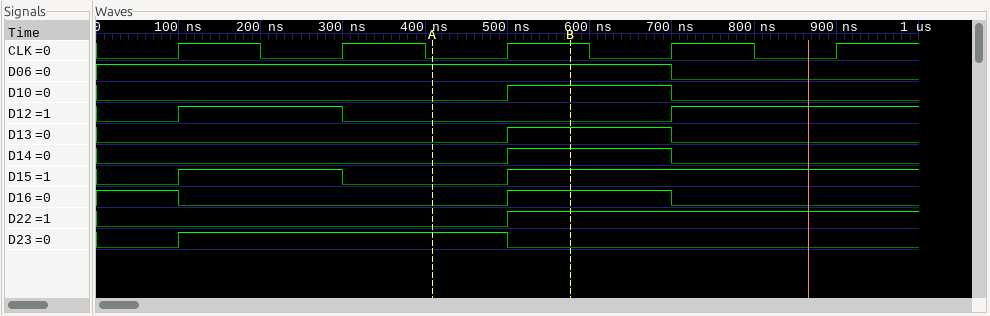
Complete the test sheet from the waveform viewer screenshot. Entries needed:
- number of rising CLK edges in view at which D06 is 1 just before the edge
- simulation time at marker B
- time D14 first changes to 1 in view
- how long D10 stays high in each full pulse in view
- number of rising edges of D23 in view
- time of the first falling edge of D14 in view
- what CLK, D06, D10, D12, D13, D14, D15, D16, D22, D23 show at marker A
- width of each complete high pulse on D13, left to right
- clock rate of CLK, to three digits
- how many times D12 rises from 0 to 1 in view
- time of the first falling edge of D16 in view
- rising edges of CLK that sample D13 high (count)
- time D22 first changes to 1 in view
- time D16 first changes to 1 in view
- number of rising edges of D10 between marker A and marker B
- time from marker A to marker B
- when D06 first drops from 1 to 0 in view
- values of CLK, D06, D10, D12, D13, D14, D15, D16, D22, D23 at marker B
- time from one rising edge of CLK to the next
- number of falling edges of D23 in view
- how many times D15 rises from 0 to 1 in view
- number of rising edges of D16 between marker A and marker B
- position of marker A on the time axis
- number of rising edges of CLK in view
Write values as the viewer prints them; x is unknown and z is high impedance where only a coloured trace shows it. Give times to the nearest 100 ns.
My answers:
4
600 ns
500 ns
200 ns
1
700 ns
CLK=0, D06=1, D10=0, D12=0, D13=0, D14=0, D15=0, D16=0, D22=0, D23=1
200 ns
5.00 MHz
2
100 ns
1
500 ns
500 ns
1
200 ns
700 ns
CLK=1, D06=1, D10=1, D12=0, D13=1, D14=1, D15=1, D16=1, D22=1, D23=0
200 ns
1
2
1
400 ns
5
